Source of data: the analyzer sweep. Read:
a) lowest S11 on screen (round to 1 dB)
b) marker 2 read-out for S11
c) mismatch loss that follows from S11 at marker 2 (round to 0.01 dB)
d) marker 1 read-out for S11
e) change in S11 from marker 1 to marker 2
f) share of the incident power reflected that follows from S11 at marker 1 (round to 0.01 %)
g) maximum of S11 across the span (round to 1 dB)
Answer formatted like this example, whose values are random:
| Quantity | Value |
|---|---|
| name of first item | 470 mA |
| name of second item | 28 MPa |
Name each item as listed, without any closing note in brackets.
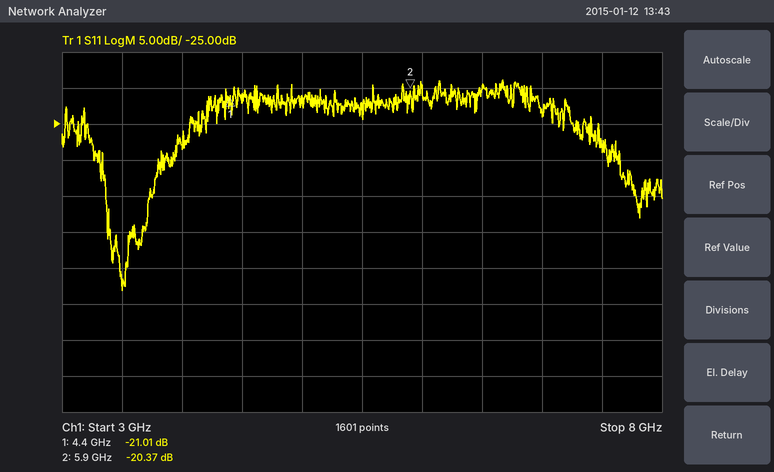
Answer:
| Quantity | Value |
|---|---|
| lowest S11 on screen | -48 dB |
| marker 2 read-out for S11 | -20.37 dB |
| mismatch loss that follows from S11 at marker 2 | 0.04 dB |
| marker 1 read-out for S11 | -21.01 dB |
| change in S11 from marker 1 to marker 2 | 0.64 dB |
| share of the incident power reflected that follows from S11 at marker 1 | 0.79 % |
| maximum of S11 across the span | -19 dB |
